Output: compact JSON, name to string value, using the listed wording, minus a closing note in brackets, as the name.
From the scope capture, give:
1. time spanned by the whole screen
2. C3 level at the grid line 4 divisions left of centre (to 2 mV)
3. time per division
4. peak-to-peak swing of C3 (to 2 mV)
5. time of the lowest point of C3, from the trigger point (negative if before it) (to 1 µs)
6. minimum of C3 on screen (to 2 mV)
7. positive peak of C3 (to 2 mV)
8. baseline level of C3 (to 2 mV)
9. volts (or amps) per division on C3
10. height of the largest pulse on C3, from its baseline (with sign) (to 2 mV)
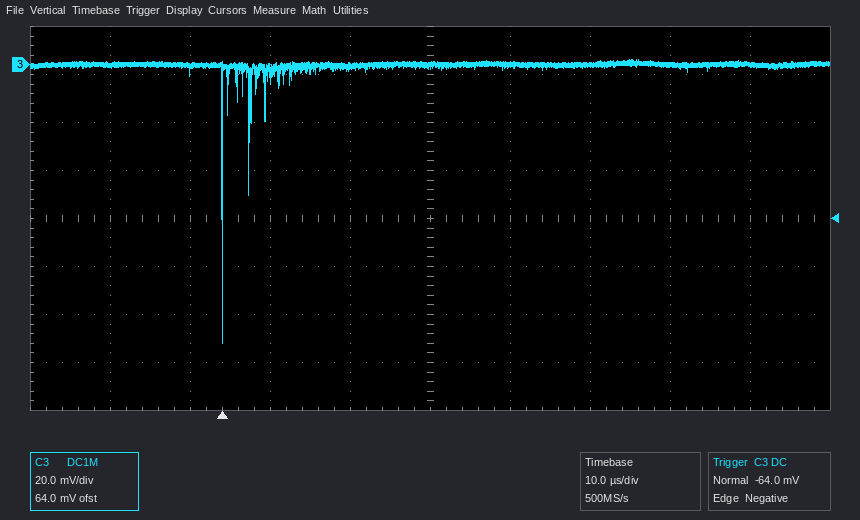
{"time spanned by the whole screen": "100 µs", "C3 level at the grid line 4 divisions left of centre": "0 mV", "time per division": "10 µs", "peak-to-peak swing of C3": "118 mV", "time of the lowest point of C3, from the trigger point (negative if before it)": "0 µs", "minimum of C3 on screen": "-116 mV", "positive peak of C3": "2 mV", "baseline level of C3": "0 mV", "volts (or amps) per division on C3": "20 mV", "height of the largest pulse on C3, from its baseline (with sign)": "-116 mV"}
